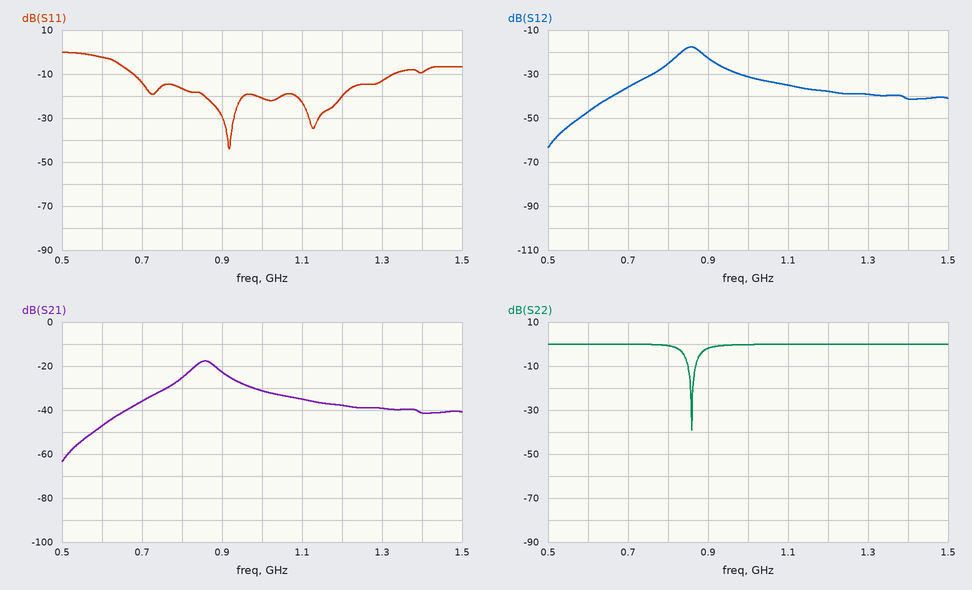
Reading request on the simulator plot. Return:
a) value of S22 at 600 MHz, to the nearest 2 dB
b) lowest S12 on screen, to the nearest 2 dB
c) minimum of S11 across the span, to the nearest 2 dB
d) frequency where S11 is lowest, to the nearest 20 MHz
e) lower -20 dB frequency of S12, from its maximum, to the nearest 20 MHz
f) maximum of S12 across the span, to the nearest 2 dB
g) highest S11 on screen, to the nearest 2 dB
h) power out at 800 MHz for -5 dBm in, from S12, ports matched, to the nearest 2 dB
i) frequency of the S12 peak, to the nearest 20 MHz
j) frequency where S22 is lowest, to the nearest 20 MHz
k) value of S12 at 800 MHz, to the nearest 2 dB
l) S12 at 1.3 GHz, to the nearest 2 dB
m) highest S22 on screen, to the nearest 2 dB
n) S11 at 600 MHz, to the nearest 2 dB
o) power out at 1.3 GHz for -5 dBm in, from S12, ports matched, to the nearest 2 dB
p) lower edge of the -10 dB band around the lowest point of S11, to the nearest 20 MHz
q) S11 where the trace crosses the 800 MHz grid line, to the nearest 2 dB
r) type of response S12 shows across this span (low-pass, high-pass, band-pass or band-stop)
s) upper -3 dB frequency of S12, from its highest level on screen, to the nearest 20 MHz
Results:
0 dB
-64 dB
-44 dB
920 MHz
680 MHz
-18 dB
0 dB
-30 dBm
860 MHz
860 MHz
-26 dB
-40 dB
0 dB
-2 dB
-44 dBm
680 MHz
-16 dB
band-pass
880 MHz
